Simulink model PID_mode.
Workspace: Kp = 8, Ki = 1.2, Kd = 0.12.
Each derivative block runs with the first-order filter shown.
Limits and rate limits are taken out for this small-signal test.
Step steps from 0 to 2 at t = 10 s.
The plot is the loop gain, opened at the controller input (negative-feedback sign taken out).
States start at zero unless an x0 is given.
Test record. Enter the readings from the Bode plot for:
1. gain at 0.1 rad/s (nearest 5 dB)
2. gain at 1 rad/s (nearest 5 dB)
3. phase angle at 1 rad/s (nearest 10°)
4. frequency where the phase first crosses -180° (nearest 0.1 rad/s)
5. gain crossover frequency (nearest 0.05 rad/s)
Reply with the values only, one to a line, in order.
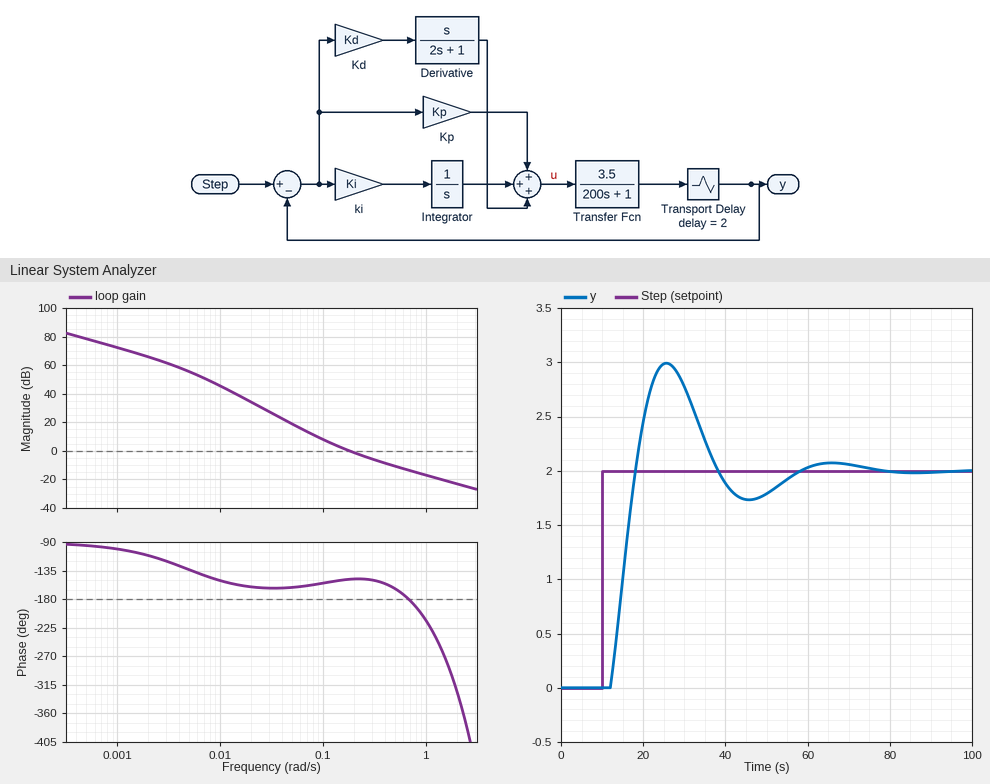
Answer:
10 dB
-15 dB
-210°
0.7 rad/s
0.20 rad/s
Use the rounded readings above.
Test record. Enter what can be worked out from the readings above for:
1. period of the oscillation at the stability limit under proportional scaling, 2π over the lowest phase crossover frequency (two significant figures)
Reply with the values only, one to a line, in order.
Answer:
9.0 s
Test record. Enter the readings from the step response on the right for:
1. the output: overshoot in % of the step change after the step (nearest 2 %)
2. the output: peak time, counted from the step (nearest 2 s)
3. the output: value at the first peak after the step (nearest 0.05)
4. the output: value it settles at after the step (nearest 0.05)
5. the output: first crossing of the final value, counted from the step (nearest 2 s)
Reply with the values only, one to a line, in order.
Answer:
50 %
16 s
3.00
2.00
8 s
